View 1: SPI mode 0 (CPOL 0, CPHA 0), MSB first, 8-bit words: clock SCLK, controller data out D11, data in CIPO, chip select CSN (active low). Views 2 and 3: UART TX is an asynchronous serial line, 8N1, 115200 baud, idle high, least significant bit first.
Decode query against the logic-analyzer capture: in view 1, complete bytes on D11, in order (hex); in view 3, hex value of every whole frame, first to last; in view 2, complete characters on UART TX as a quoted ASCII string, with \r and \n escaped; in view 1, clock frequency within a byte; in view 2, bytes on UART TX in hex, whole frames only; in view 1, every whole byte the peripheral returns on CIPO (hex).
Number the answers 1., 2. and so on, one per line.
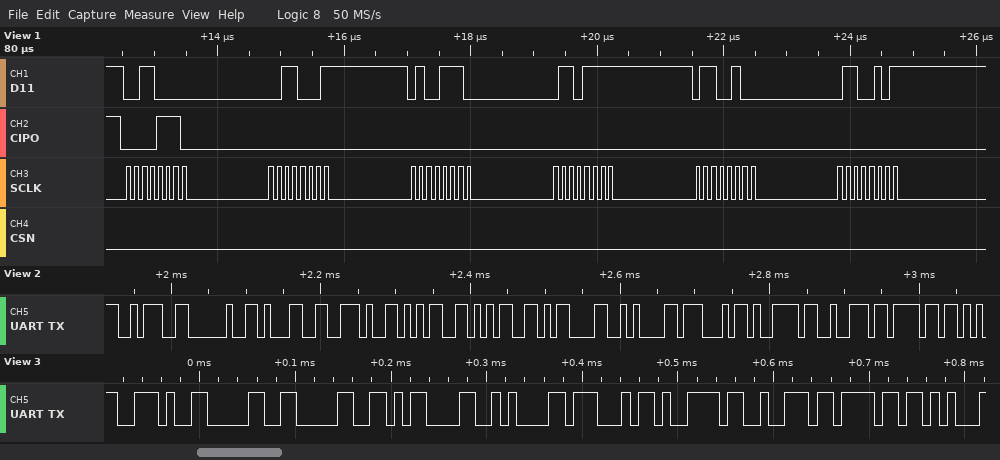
1. 30 31 4E 6F 64 65
2. 2E 30 30 0D 0A 47 79 72 6F
3. ": 1.55\r\nGyro"
4. 8 MHz
5. 3A 20 31 2E 35 35 0D 0A 47 79 72 6F
6. 0E 00 00 00 00 00
